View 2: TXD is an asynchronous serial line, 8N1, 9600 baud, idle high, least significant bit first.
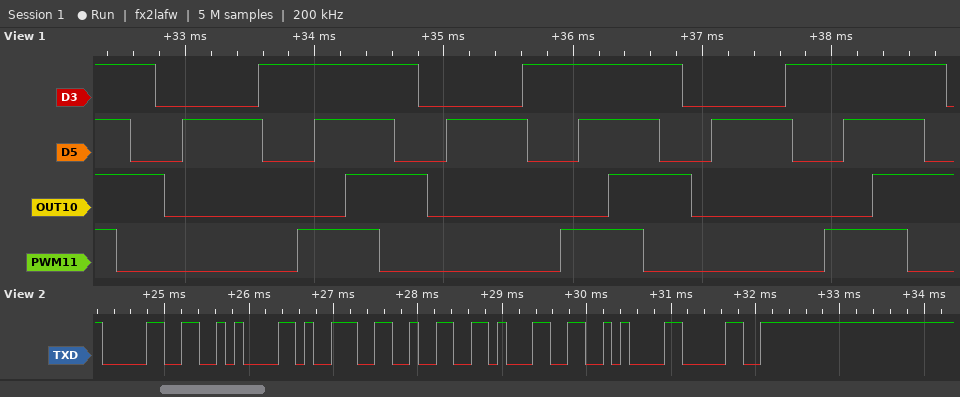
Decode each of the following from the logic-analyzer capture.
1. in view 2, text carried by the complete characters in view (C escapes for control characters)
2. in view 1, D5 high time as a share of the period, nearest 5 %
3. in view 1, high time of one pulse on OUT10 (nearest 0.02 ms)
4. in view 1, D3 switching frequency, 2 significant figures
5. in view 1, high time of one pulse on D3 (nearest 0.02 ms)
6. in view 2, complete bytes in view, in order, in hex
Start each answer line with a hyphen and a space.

- "0\n921\n0"
- 60 %
- 0.64 ms
- 490 Hz
- 1.24 ms
- 30 0A 39 32 31 0A 30
